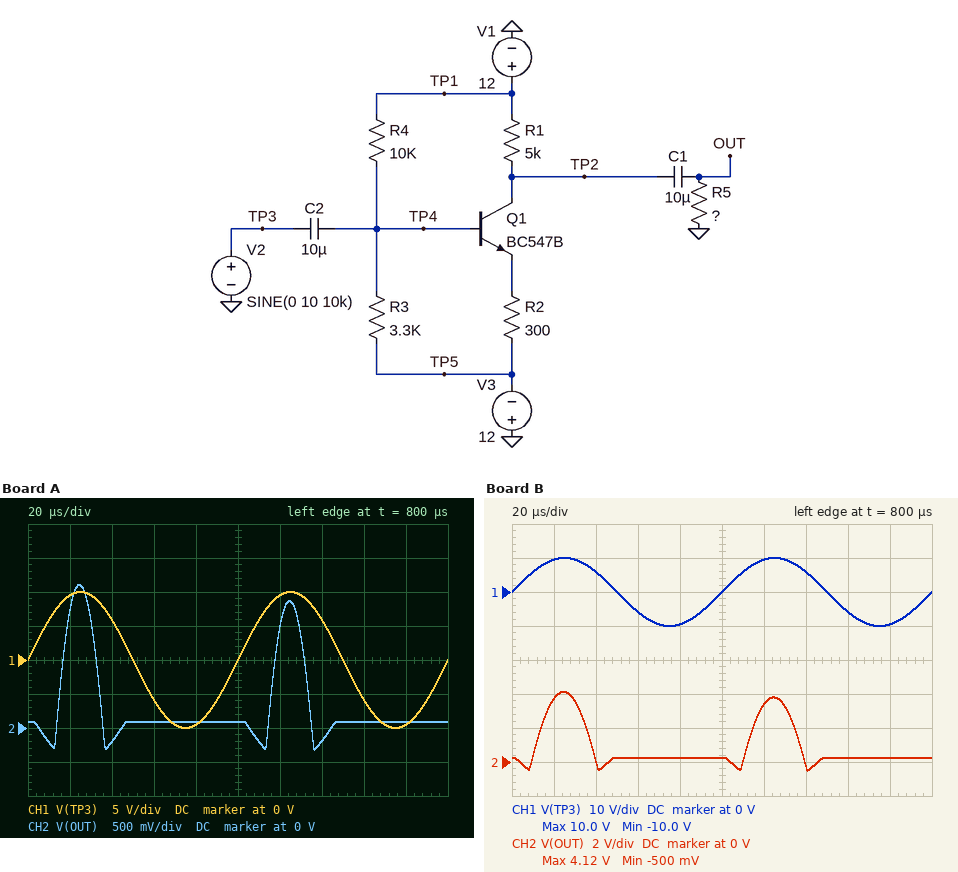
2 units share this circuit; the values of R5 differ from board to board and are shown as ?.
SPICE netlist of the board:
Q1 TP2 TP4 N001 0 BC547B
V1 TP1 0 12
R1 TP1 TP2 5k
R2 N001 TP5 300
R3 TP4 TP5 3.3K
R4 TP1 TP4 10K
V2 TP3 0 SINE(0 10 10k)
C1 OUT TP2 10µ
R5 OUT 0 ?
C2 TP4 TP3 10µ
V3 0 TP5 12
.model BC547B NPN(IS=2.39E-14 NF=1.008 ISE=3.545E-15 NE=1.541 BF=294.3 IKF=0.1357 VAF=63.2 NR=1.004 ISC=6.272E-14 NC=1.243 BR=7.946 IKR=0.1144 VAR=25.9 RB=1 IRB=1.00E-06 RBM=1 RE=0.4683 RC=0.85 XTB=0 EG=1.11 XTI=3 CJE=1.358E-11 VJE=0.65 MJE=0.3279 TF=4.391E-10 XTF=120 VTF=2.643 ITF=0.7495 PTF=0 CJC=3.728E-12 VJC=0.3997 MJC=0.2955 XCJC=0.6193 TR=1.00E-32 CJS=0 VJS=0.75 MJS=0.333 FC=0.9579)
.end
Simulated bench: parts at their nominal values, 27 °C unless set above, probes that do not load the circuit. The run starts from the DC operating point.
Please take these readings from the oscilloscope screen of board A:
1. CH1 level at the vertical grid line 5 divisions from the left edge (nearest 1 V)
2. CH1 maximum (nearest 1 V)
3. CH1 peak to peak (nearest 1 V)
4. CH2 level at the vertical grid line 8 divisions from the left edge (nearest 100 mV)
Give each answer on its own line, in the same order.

0 V
10 V
20 V
100 mV
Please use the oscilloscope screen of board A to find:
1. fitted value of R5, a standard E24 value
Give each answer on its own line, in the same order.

24 Ω
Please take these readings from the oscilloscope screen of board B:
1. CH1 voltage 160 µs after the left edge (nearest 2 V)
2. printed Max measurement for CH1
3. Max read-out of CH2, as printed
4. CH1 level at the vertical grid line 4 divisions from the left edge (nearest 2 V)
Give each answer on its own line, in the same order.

-6 V
10.0 V
4.12 V
-10 V
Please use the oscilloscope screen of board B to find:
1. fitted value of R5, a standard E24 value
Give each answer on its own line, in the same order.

56 Ω
